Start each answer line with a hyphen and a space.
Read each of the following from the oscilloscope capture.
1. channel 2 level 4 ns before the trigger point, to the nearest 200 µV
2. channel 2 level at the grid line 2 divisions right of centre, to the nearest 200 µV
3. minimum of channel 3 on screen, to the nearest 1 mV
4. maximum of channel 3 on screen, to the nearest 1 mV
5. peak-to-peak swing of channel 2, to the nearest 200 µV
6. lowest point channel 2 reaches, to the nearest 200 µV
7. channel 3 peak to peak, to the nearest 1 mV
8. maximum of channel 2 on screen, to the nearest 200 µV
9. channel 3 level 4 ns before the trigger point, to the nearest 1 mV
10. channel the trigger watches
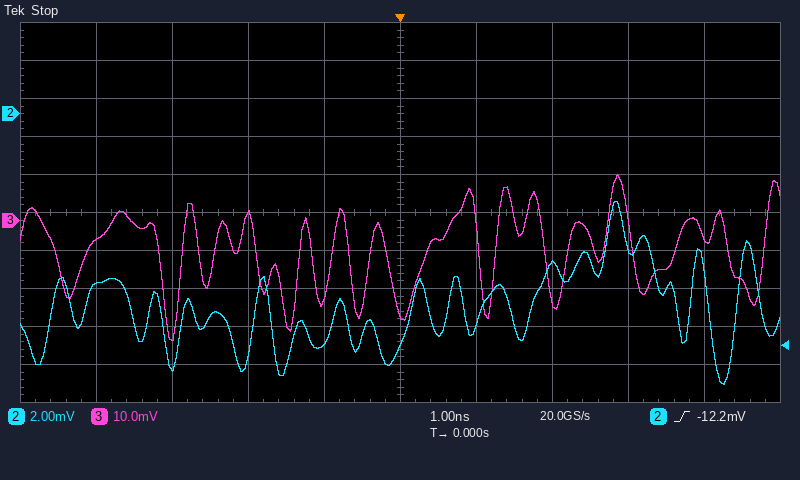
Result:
- -9.0 mV
- -8.0 mV
- -32 mV
- 12 mV
- 9.6 mV
- -14.2 mV
- 44 mV
- -4.6 mV
- -5 mV
- channel 2
